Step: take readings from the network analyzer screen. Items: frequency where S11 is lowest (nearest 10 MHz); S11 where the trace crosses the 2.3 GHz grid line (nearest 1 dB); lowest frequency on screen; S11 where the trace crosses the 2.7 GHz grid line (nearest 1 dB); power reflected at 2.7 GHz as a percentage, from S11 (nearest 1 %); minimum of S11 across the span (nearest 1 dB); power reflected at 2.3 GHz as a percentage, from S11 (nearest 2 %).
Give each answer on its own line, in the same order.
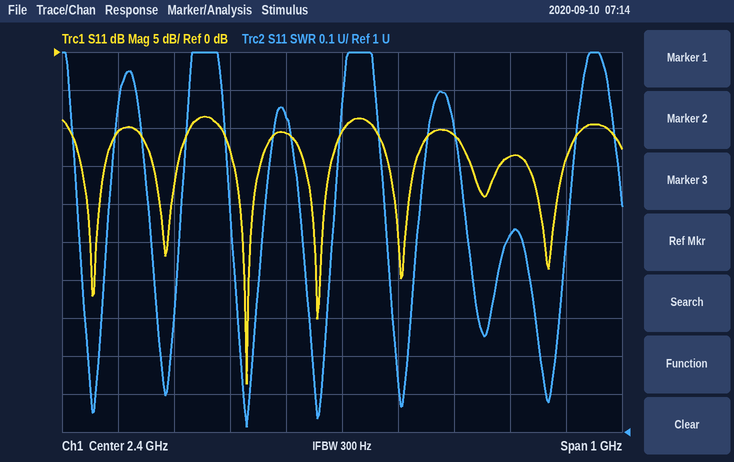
2.23 GHz
-11 dB
1.9 GHz
-14 dB
4 %
-44 dB
8 %
